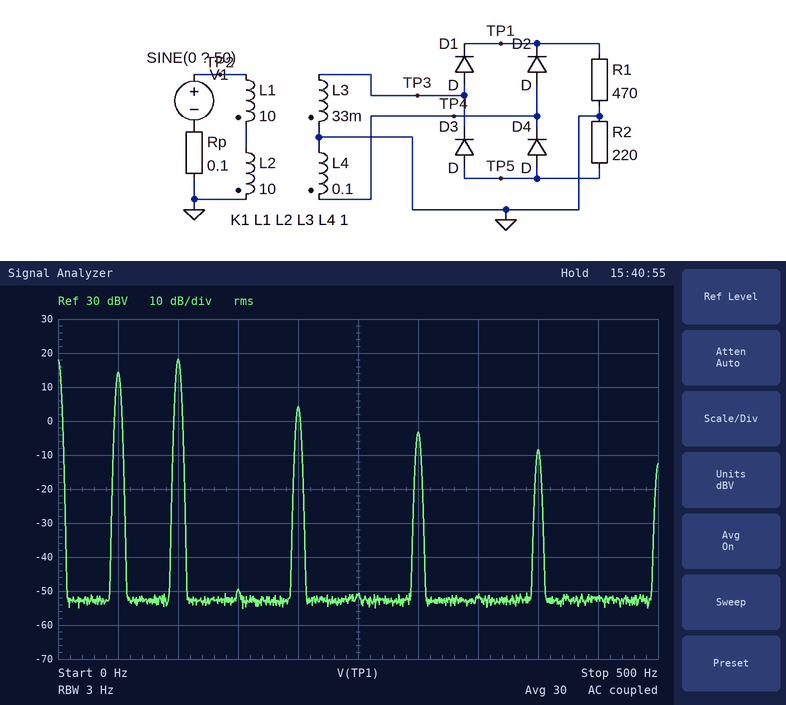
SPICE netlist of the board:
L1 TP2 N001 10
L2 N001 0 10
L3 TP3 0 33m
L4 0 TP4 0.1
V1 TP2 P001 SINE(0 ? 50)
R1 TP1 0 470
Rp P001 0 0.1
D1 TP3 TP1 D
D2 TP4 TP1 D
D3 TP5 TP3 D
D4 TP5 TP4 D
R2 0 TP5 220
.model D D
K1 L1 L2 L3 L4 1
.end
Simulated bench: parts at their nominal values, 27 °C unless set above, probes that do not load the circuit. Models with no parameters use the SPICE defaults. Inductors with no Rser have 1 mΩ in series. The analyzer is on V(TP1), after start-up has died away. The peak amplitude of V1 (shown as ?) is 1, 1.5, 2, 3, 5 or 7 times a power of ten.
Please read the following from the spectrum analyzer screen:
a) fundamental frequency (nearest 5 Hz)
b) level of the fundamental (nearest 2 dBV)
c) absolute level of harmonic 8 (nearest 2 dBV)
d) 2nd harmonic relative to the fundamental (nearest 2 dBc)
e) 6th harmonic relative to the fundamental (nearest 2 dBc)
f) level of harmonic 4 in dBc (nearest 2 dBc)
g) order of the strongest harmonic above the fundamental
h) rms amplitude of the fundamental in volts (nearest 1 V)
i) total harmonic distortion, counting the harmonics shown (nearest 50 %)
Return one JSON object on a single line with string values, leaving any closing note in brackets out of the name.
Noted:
{"fundamental frequency": "50 Hz", "level of the fundamental": "14 dBV", "absolute level of harmonic 8": "-8 dBV", "2nd harmonic relative to the fundamental": "4 dBc", "6th harmonic relative to the fundamental": "-18 dBc", "level of harmonic 4 in dBc": "-10 dBc", "order of the strongest harmonic above the fundamental": "2", "rms amplitude of the fundamental in volts": "5 V", "total harmonic distortion, counting the harmonics shown": "150 %"}
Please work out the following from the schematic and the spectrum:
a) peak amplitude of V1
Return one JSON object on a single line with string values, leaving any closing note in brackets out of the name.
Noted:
{"peak amplitude of V1": "700 V"}
